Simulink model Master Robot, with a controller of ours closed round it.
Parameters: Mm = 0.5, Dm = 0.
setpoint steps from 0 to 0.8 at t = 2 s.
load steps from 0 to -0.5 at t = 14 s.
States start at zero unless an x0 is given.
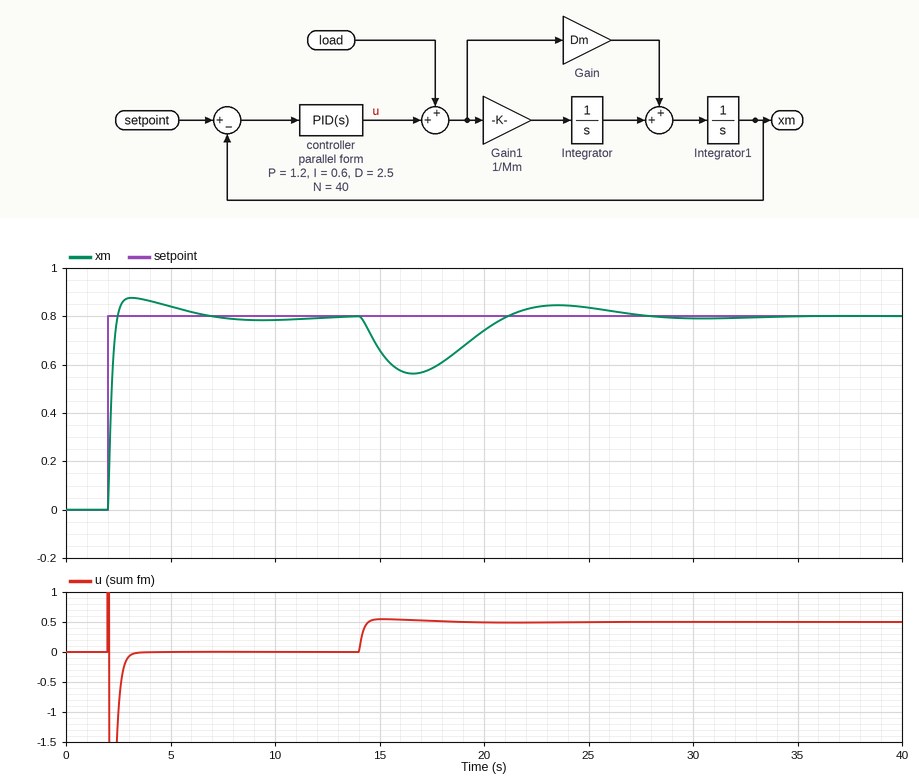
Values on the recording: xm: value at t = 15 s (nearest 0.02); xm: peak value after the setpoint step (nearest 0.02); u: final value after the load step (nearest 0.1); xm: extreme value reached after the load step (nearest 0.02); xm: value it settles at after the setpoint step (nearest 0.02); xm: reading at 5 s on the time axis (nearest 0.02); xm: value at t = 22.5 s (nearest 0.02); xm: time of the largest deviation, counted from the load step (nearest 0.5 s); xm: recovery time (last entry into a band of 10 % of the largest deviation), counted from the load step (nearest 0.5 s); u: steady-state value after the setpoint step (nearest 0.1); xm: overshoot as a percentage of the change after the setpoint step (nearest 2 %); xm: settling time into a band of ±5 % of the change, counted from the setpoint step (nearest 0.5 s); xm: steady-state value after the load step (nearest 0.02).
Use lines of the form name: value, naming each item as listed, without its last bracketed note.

xm: value at t = 15 s: 0.66
xm: peak value after the setpoint step: 0.88
u: final value after the load step: 0.5
xm: extreme value reached after the load step: 0.56
xm: value it settles at after the setpoint step: 0.80
xm: reading at 5 s on the time axis: 0.84
xm: value at t = 22.5 s: 0.84
xm: time of the largest deviation, counted from the load step: 2.5 s
xm: recovery time (last entry into a band of 10 % of the largest deviation), counted from the load step: 12.0 s
u: steady-state value after the setpoint step: 0.0
xm: overshoot as a percentage of the change after the setpoint step: 10 %
xm: settling time into a band of ±5 % of the change, counted from the setpoint step: 3.0 s
xm: steady-state value after the load step: 0.80
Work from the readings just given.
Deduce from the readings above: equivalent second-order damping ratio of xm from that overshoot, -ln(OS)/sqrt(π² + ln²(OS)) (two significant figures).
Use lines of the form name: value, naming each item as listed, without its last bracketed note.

equivalent second-order damping ratio of xm from that overshoot, -ln(OS)/sqrt(π² + ln²(OS)): 0.59
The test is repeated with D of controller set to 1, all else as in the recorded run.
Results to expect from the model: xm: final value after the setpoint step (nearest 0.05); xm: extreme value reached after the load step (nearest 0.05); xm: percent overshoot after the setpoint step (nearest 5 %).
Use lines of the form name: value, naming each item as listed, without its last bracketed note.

xm: final value after the setpoint step: 0.80
xm: extreme value reached after the load step: 0.45
xm: percent overshoot after the setpoint step: 35 %
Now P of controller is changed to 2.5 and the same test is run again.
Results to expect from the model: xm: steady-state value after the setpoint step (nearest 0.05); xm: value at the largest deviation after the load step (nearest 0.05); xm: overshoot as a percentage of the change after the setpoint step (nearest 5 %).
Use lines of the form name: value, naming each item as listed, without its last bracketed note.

xm: steady-state value after the setpoint step: 0.80
xm: value at the largest deviation after the load step: 0.65
xm: overshoot as a percentage of the change after the setpoint step: 15 %
